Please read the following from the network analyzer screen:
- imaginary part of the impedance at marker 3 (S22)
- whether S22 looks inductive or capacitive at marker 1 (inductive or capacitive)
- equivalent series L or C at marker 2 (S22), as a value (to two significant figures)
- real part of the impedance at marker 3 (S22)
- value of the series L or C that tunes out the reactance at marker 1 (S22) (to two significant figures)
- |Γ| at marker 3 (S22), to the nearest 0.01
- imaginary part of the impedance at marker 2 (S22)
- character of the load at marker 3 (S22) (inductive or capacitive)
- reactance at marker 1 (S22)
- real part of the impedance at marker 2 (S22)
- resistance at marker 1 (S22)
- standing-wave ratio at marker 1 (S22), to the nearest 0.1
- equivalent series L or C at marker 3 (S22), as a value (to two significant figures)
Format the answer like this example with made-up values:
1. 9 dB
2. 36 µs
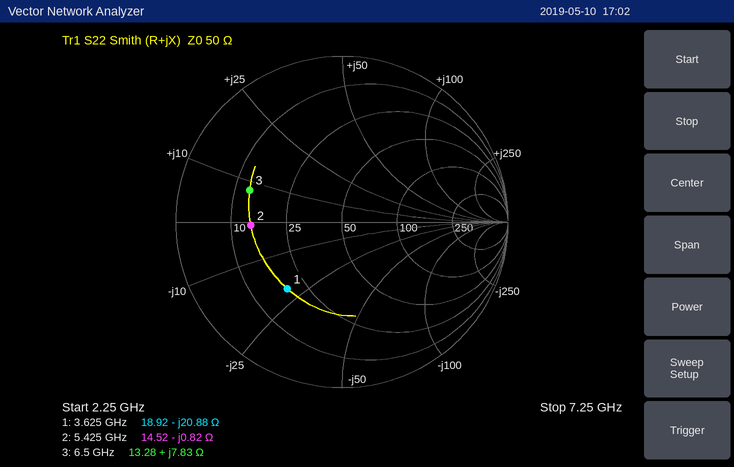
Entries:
1. +7.83 Ω
2. capacitive
3. 36 pF
4. 13.28 Ω
5. 920 pH
6. 0.59
7. -0.82 Ω
8. inductive
9. -20.88 Ω
10. 14.52 Ω
11. 18.92 Ω
12. 3.2
13. 190 pH
